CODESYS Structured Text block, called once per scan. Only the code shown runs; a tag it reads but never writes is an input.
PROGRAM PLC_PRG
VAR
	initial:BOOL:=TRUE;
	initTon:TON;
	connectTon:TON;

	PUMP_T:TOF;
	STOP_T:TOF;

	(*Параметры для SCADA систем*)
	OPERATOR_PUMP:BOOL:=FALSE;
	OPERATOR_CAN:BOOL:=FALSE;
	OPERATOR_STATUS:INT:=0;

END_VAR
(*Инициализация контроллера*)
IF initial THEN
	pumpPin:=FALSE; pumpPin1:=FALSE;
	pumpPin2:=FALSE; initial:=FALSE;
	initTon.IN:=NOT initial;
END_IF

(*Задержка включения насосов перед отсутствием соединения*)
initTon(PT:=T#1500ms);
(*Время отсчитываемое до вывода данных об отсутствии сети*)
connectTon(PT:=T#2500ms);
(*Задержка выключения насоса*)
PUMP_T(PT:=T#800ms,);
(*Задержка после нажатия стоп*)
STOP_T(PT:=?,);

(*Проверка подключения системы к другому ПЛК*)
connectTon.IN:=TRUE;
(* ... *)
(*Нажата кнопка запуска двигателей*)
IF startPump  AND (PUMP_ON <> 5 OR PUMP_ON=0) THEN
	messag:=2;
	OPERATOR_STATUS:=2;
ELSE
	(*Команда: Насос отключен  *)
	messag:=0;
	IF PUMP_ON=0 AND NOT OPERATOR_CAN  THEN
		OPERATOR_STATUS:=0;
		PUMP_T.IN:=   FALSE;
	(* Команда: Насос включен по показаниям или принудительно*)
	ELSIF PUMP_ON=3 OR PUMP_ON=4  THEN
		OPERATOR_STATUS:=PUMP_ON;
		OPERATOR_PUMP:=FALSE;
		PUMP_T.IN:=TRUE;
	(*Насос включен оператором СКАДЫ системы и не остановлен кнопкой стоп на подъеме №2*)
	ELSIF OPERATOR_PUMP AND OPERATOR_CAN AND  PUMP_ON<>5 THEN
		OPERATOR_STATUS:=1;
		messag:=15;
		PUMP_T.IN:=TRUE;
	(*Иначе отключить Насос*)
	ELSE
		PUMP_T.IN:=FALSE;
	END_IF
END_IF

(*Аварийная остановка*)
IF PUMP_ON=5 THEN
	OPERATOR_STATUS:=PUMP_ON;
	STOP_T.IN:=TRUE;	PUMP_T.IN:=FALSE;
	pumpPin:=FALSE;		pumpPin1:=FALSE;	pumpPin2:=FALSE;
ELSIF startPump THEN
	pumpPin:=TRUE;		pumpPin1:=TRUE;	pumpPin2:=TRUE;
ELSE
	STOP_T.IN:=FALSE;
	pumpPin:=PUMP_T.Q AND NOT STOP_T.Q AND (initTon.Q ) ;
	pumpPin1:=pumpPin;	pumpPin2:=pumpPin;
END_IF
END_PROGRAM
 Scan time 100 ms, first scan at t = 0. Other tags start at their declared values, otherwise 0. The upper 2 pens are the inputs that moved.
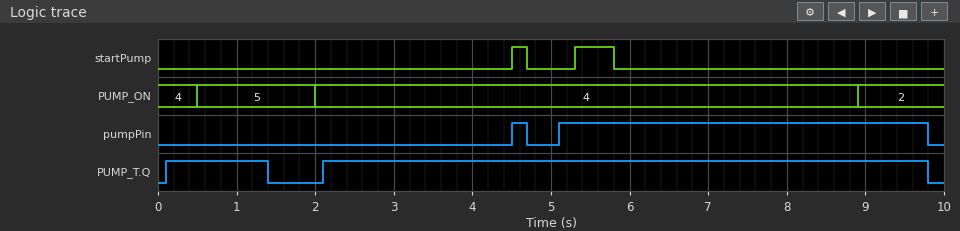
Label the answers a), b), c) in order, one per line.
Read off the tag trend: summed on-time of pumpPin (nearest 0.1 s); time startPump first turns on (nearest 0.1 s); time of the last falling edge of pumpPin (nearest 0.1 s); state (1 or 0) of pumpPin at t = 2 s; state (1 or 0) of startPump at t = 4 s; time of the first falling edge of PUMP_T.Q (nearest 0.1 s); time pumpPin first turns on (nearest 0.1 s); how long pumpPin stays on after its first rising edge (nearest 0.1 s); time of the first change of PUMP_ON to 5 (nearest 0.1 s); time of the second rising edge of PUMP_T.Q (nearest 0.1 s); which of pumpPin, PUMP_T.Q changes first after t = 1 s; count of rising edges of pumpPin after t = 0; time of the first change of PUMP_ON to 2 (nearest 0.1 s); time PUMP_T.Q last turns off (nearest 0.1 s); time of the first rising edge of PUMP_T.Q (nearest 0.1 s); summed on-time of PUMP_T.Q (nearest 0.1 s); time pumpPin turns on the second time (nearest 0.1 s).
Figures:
a) 4.9 s
b) 4.5 s
c) 9.8 s
d) 0
e) 0
f) 1.4 s
g) 4.5 s
h) 0.2 s
i) 0.5 s
j) 2.1 s
k) PUMP_T.Q
l) 2
m) 8.9 s
n) 9.8 s
o) 0.1 s
p) 9.0 s
q) 5.1 s
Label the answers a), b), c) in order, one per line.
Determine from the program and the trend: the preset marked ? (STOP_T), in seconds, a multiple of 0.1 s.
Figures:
a) 3.0 s
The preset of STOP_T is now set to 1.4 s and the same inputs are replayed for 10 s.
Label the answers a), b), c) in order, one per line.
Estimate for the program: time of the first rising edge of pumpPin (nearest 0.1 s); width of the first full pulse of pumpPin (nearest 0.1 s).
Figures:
a) 3.5 s
b) 6.3 s
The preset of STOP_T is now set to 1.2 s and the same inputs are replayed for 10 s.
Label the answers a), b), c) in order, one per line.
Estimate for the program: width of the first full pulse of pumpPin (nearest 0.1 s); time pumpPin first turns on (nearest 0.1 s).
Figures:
a) 6.5 s
b) 3.3 s
